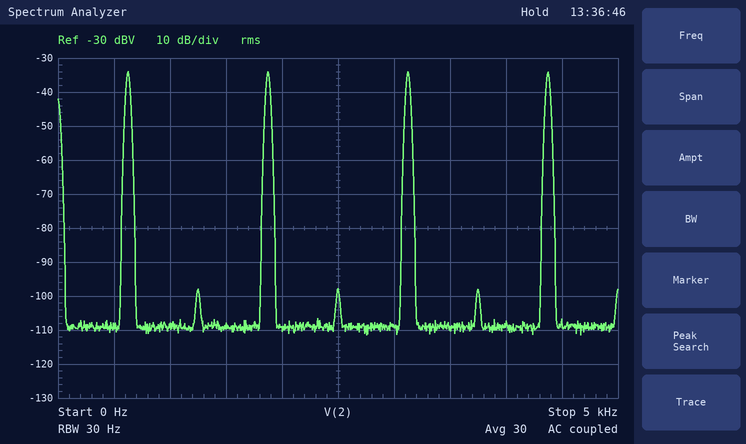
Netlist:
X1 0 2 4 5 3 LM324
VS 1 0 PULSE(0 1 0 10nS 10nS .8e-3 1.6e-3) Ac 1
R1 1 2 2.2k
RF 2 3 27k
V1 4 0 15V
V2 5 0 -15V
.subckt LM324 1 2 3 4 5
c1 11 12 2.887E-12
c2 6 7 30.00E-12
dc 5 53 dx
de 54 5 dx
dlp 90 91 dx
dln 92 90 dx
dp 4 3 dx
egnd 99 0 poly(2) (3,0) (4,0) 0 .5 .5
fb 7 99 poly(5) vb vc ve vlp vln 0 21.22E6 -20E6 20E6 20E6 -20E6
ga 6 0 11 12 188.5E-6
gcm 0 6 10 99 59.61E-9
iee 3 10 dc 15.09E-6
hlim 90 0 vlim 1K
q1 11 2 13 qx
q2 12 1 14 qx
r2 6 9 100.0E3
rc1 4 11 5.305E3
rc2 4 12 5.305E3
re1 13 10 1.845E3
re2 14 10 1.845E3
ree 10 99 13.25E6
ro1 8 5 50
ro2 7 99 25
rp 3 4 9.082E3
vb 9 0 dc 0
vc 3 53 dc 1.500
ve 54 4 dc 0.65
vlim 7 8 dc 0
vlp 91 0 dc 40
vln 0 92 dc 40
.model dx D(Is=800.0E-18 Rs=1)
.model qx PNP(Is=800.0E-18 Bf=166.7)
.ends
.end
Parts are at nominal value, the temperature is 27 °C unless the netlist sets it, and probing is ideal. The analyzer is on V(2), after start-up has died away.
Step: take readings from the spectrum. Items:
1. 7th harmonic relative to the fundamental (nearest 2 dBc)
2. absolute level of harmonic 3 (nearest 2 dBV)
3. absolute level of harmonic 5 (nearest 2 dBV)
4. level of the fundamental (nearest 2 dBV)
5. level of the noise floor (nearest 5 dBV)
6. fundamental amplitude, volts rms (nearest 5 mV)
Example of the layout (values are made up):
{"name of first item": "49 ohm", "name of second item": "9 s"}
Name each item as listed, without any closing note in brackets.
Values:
{"7th harmonic relative to the fundamental": "0 dBc", "absolute level of harmonic 3": "-34 dBV", "absolute level of harmonic 5": "-34 dBV", "level of the fundamental": "-34 dBV", "level of the noise floor": "-110 dBV", "fundamental amplitude, volts rms": "20 mV"}
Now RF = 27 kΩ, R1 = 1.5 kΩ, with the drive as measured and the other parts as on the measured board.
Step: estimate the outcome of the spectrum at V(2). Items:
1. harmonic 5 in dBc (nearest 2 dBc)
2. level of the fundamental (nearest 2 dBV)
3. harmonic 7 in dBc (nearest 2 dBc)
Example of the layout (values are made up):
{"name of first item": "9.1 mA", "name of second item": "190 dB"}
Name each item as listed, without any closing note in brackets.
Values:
{"harmonic 5 in dBc": "-8 dBc", "level of the fundamental": "-22 dBV", "harmonic 7 in dBc": "-10 dBc"}
